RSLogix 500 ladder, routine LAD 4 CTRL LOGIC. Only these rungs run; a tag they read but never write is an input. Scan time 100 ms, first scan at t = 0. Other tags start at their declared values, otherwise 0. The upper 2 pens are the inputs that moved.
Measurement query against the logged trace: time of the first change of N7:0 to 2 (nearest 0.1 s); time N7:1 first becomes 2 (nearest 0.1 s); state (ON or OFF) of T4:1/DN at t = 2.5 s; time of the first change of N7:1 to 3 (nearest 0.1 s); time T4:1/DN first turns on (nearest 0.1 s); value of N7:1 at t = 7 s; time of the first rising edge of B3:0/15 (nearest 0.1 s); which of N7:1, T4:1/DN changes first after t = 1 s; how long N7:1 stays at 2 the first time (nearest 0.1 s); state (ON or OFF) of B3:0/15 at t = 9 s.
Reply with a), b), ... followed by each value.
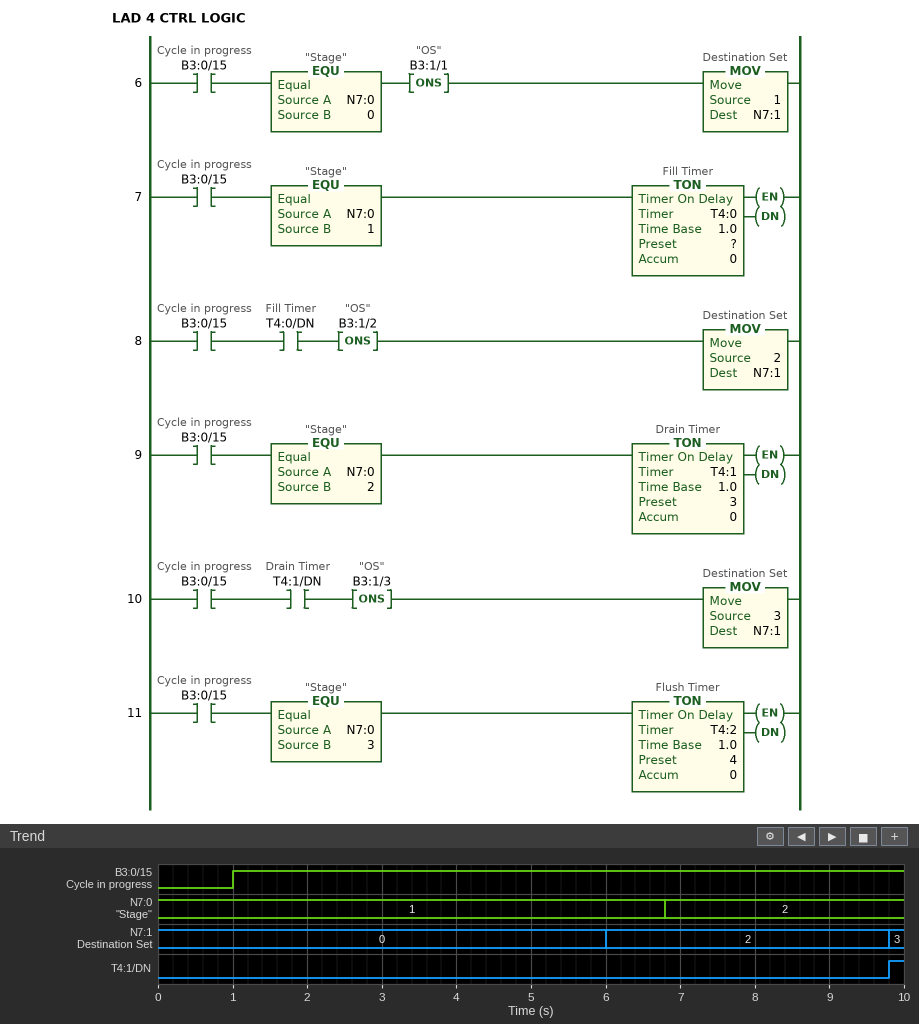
a) 6.8 s
b) 6.0 s
c) OFF
d) 9.8 s
e) 9.8 s
f) 2
g) 1.0 s
h) N7:1
i) 3.8 s
j) ON
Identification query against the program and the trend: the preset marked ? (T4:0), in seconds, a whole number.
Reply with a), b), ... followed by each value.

a) 5 s
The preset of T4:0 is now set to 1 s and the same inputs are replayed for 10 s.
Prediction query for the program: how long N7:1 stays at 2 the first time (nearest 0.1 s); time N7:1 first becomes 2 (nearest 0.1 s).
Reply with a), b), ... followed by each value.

a) 7.8 s
b) 2.0 s
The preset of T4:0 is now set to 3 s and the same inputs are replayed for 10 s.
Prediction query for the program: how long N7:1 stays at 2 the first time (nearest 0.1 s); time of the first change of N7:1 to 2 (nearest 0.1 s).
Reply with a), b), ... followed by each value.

a) 5.8 s
b) 4.0 s
